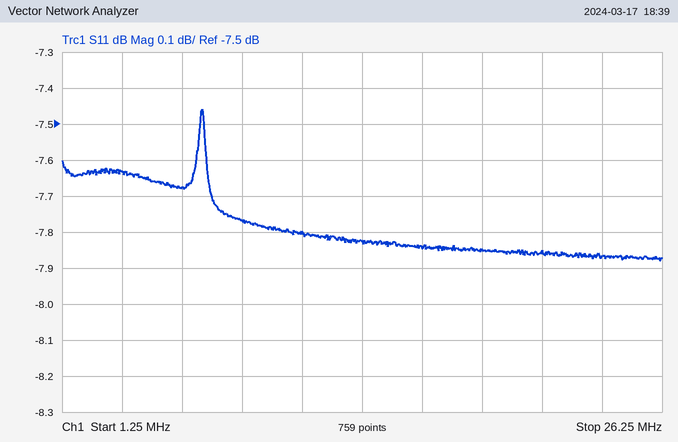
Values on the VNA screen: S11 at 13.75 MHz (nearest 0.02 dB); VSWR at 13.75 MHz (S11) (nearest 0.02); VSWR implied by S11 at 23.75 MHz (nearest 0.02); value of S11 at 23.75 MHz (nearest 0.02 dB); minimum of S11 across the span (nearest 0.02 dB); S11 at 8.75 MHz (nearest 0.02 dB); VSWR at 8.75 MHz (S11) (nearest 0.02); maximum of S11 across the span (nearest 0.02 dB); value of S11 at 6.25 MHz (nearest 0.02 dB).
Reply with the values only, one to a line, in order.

-7.82 dB
2.36
2.36
-7.86 dB
-7.88 dB
-7.76 dB
2.38
-7.46 dB
-7.68 dB
